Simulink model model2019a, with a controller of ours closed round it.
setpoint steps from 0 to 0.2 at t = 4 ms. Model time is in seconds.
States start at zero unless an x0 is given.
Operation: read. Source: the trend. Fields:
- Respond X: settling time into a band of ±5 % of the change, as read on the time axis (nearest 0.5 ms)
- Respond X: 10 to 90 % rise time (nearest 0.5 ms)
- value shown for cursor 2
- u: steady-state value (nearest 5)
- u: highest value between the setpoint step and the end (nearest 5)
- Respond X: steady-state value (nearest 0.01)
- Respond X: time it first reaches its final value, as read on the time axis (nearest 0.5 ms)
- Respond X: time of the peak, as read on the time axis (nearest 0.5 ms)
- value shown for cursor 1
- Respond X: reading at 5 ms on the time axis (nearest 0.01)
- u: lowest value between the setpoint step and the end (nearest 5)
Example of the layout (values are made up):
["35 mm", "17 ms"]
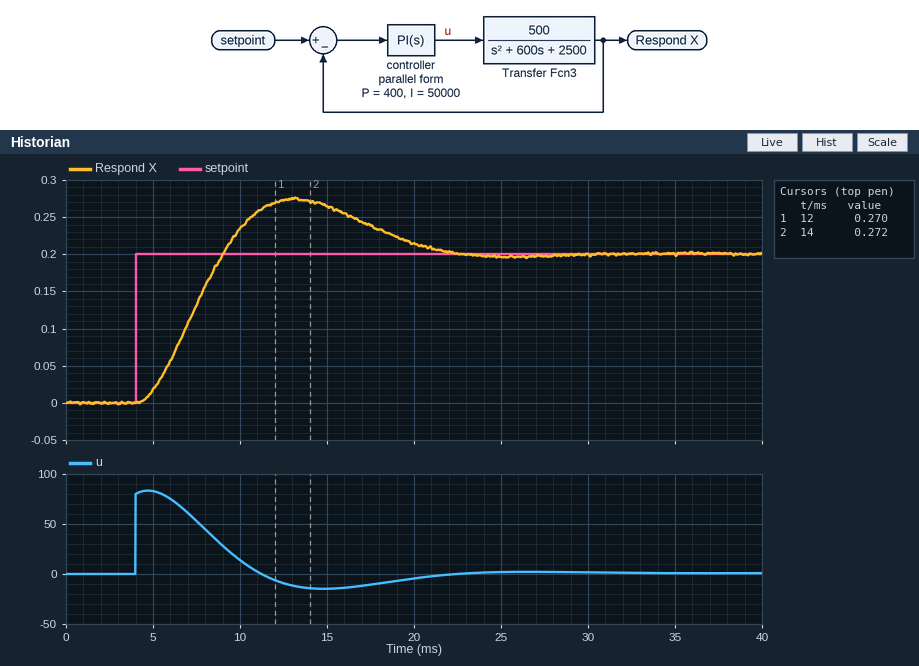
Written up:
["20.5 ms", "3.5 ms", "0.272", "0", "85", "0.20", "9.0 ms", "13.0 ms", "0.270", "0.02", "-15"]
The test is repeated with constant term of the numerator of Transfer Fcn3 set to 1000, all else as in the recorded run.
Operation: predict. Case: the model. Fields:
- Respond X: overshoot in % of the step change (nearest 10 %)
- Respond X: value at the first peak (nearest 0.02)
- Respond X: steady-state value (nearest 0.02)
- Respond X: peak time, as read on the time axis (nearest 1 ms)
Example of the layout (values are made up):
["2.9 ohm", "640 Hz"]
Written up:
["40 %", "0.28", "0.20", "10 ms"]
